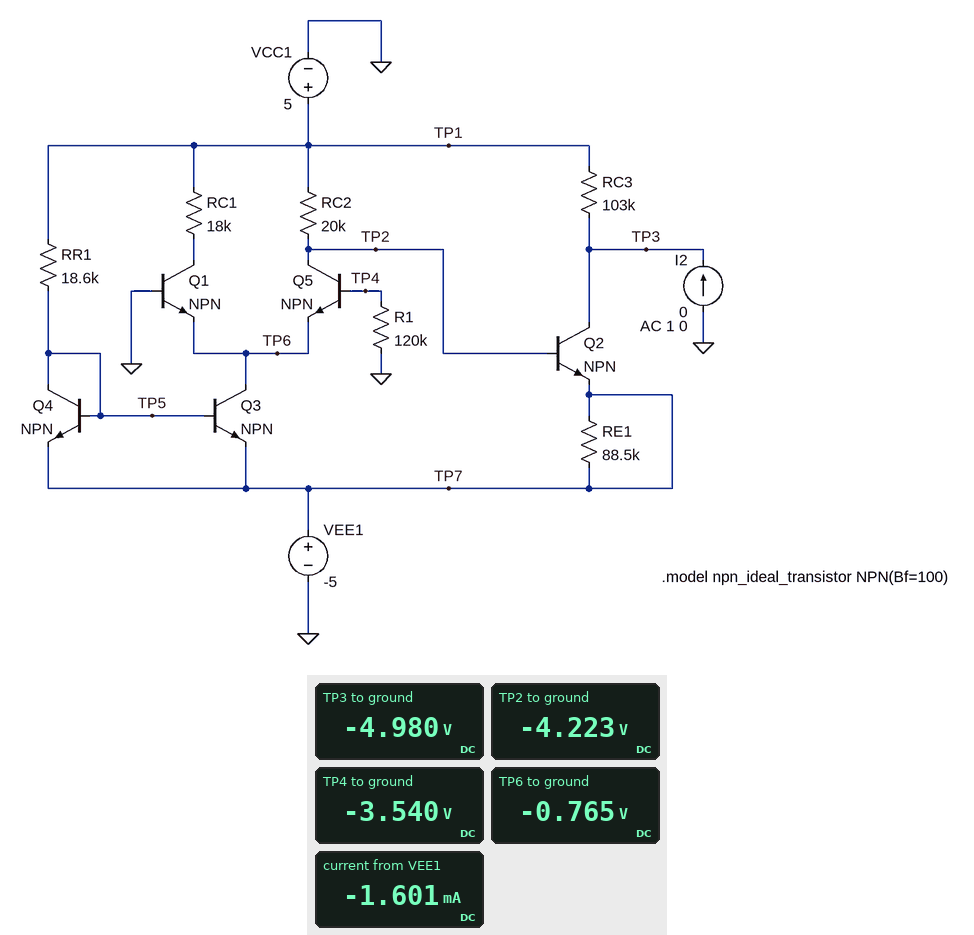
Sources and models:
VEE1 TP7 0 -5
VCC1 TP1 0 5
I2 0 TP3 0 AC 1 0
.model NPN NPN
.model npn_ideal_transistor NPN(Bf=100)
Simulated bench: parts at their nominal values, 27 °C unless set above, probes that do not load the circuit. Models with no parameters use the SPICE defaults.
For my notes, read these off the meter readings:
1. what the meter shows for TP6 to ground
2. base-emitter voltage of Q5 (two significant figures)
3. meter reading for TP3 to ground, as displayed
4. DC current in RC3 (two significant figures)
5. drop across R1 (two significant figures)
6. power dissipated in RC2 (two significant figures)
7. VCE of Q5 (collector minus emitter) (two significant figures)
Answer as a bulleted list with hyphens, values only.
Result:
- -0.765 V
- -2.8 V
- -4.980 V
- 97 µA
- 3.5 V
- 4.3 mW
- -3.5 V
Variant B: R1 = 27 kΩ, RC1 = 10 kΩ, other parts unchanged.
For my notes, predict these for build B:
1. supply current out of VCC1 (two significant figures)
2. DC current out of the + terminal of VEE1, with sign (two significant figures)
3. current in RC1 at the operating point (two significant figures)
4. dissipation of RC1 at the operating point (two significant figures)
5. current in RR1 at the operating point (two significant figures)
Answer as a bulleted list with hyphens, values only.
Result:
- 1.6 mA
- -1.8 mA
- 570 µA
- 3.2 mW
- 500 µA
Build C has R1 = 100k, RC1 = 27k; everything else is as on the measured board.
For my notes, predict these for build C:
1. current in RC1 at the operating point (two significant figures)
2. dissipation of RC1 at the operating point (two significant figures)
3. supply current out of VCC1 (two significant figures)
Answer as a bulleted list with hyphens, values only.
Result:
- 210 µA
- 1.2 mW
- 1.3 mA
